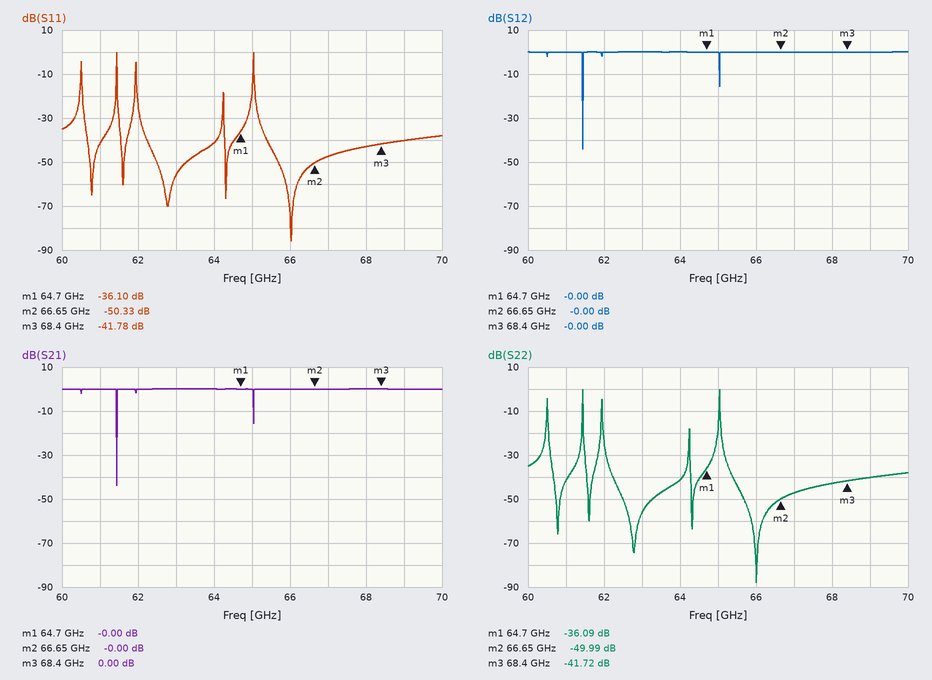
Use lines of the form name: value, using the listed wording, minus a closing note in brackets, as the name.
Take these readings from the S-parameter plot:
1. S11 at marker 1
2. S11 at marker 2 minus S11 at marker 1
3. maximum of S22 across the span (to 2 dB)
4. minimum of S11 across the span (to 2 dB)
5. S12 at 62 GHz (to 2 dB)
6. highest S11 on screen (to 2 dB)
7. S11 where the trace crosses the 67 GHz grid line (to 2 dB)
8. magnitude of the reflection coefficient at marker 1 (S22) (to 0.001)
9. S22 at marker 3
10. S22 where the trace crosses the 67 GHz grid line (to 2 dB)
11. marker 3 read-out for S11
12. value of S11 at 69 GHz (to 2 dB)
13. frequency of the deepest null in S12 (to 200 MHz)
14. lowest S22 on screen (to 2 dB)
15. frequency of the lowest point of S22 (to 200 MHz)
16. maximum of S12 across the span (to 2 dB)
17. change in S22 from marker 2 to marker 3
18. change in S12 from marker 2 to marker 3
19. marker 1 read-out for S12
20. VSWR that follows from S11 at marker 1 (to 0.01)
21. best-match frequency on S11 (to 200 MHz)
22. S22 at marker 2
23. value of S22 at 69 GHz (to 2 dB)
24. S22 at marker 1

S11 at marker 1: -36.10 dB
S11 at marker 2 minus S11 at marker 1: -14.23 dB
maximum of S22 across the span: 0 dB
minimum of S11 across the span: -86 dB
S12 at 62 GHz: 0 dB
highest S11 on screen: 0 dB
S11 where the trace crosses the 67 GHz grid line: -48 dB
magnitude of the reflection coefficient at marker 1 (S22): 0.016
S22 at marker 3: -41.72 dB
S22 where the trace crosses the 67 GHz grid line: -48 dB
marker 3 read-out for S11: -41.78 dB
value of S11 at 69 GHz: -40 dB
frequency of the deepest null in S12: 61.4 GHz
lowest S22 on screen: -88 dB
frequency of the lowest point of S22: 66.0 GHz
maximum of S12 across the span: 0 dB
change in S22 from marker 2 to marker 3: 8.27 dB
change in S12 from marker 2 to marker 3: 0.00 dB
marker 1 read-out for S12: -0.00 dB
VSWR that follows from S11 at marker 1: 1.03
best-match frequency on S11: 66.0 GHz
S22 at marker 2: -49.99 dB
value of S22 at 69 GHz: -40 dB
S22 at marker 1: -36.09 dB
